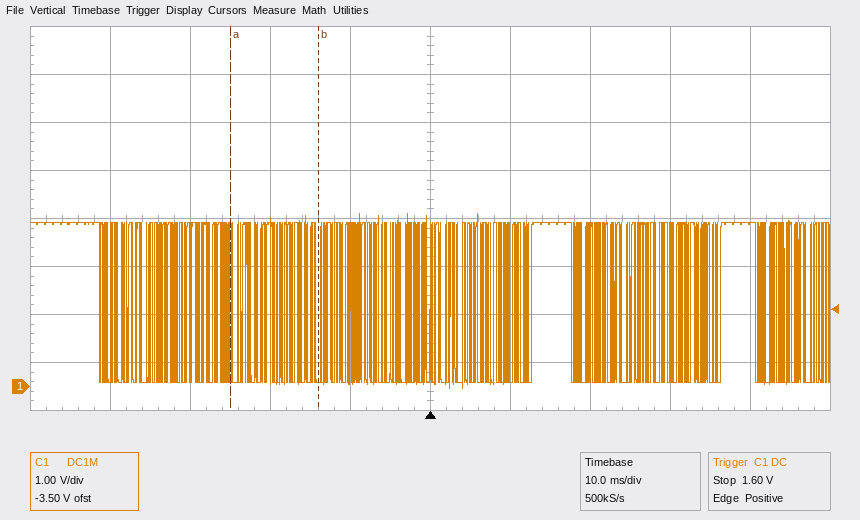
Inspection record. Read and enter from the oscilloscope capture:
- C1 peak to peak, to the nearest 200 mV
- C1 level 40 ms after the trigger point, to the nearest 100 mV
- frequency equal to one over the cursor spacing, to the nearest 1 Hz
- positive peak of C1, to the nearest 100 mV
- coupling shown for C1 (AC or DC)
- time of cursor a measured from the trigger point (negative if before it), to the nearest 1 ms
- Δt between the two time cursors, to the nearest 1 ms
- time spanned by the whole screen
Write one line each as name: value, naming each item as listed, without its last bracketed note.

C1 peak to peak, to the nearest 200 mV: 3.6 V
C1 level 40 ms after the trigger point, to the nearest 100 mV: 3.4 V
frequency equal to one over the cursor spacing, to the nearest 1 Hz: 91 Hz
positive peak of C1, to the nearest 100 mV: 3.6 V
coupling shown for C1: DC
time of cursor a measured from the trigger point (negative if before it), to the nearest 1 ms: -25 ms
Δt between the two time cursors, to the nearest 1 ms: 11 ms
time spanned by the whole screen: 100 ms
